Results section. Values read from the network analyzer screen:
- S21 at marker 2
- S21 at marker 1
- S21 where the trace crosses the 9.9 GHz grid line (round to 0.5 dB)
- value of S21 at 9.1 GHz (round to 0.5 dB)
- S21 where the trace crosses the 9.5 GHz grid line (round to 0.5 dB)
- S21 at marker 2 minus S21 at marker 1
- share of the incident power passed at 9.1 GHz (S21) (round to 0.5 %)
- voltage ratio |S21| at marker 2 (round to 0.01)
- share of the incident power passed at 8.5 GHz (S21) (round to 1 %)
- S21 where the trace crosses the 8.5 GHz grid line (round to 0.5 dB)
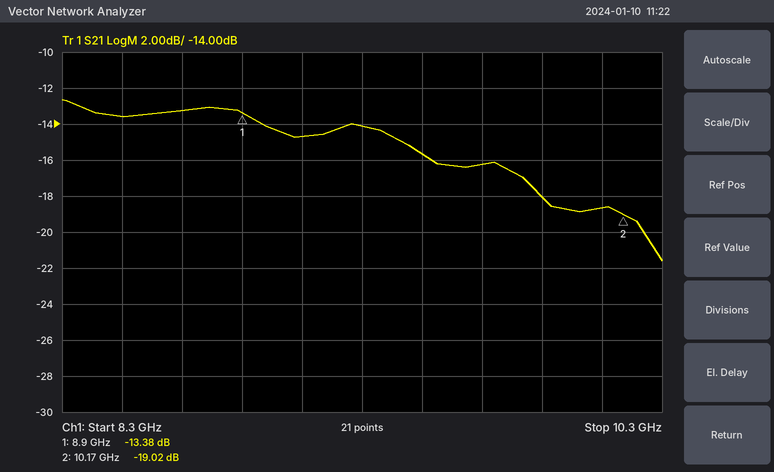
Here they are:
-19.02 dB
-13.38 dB
-18.0 dB
-14.5 dB
-15.5 dB
-5.64 dB
3.5 %
0.11
4 %
-13.5 dB
